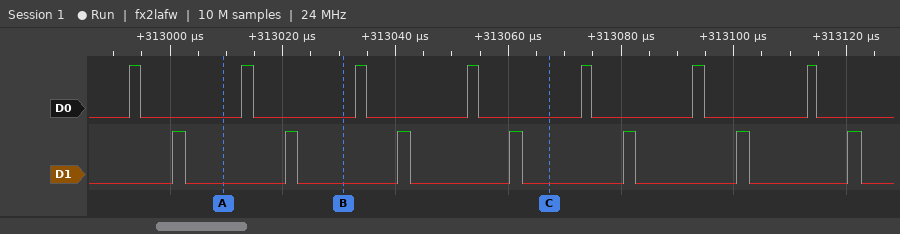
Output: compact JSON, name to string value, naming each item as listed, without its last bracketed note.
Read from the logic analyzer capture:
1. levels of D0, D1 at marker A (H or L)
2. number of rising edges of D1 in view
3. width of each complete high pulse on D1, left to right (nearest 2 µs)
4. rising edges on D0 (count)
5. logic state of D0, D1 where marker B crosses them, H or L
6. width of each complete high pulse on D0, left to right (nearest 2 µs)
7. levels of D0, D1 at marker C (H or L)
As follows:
{"levels of D0, D1 at marker A": "D0=L, D1=L", "number of rising edges of D1 in view": "7", "width of each complete high pulse on D1, left to right": "2 µs, 2 µs, 2 µs, 2 µs, 2 µs, 2 µs, 2 µs", "rising edges on D0": "7", "logic state of D0, D1 where marker B crosses them, H or L": "D0=L, D1=L", "width of each complete high pulse on D0, left to right": "2 µs, 2 µs, 2 µs, 2 µs, 2 µs, 2 µs, 2 µs", "levels of D0, D1 at marker C": "D0=L, D1=L"}
